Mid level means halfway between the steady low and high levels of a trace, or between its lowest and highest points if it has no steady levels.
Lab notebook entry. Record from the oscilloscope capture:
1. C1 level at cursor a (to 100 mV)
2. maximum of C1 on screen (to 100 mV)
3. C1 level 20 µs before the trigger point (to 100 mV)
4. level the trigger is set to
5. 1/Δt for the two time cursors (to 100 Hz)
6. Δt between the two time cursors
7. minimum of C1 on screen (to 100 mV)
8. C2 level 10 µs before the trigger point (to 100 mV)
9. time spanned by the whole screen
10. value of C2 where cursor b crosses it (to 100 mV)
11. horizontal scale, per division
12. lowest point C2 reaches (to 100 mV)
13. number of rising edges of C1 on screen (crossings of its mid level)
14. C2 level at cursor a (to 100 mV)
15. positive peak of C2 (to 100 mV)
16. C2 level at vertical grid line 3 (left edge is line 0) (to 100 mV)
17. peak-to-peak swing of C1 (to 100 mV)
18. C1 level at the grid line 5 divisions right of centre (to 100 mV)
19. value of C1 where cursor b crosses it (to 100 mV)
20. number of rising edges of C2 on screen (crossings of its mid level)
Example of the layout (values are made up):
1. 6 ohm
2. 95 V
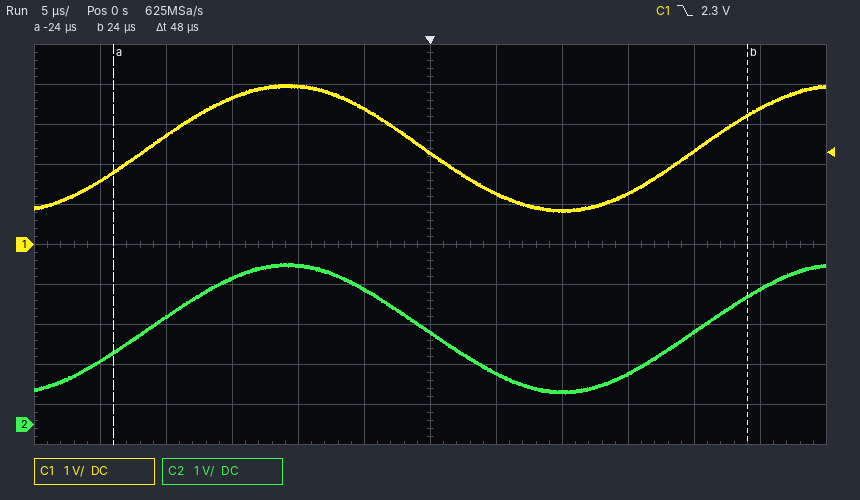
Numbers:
1. 1.8 V
2. 4.0 V
3. 2.7 V
4. 2.3 V
5. 20.8 kHz
6. 48 µs
7. 800 mV
8. 4.0 V
9. 60 µs
10. 3.2 V
11. 5 µs
12. 800 mV
13. 2
14. 1.8 V
15. 4.0 V
16. 3.7 V
17. 3.2 V
18. 3.4 V
19. 3.2 V
20. 2
